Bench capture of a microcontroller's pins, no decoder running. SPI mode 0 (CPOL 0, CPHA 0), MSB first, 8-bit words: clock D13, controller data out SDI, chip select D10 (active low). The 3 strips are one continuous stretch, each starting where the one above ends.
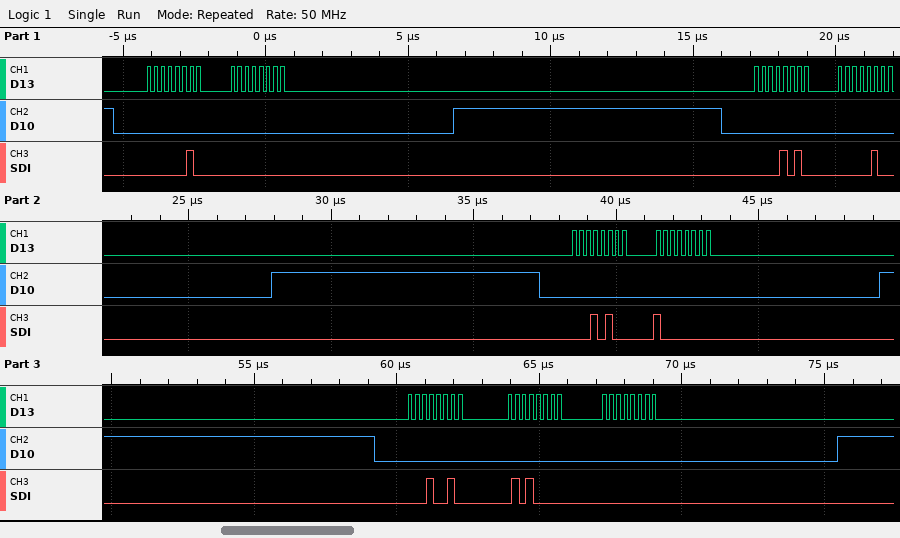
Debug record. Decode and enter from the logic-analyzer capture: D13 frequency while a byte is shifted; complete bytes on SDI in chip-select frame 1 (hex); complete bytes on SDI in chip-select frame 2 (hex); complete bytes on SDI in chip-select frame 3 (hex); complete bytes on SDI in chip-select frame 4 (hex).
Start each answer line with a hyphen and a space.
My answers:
- 4 MHz
- 0x02 0x00
- 0x0A 0x04
- 0x14 0x80
- 0x12 0x50 0x00
